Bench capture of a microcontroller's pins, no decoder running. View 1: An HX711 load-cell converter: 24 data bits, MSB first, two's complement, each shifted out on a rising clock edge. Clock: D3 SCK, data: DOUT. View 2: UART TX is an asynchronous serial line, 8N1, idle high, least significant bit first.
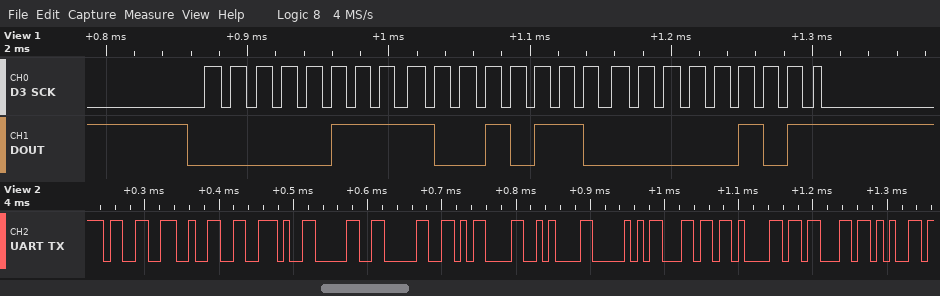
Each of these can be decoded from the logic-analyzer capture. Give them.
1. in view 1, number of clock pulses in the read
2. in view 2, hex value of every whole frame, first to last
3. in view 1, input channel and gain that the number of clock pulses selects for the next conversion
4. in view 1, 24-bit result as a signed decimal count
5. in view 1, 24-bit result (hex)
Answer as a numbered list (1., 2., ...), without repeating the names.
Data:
1. 25
2. 0x33 0x32 0x2E 0x30 0x30 0x0D 0x0A 0x50 0x6C 0x61 0x63 0x65
3. channel A, gain 128
4. 497157
5. 0x079605
